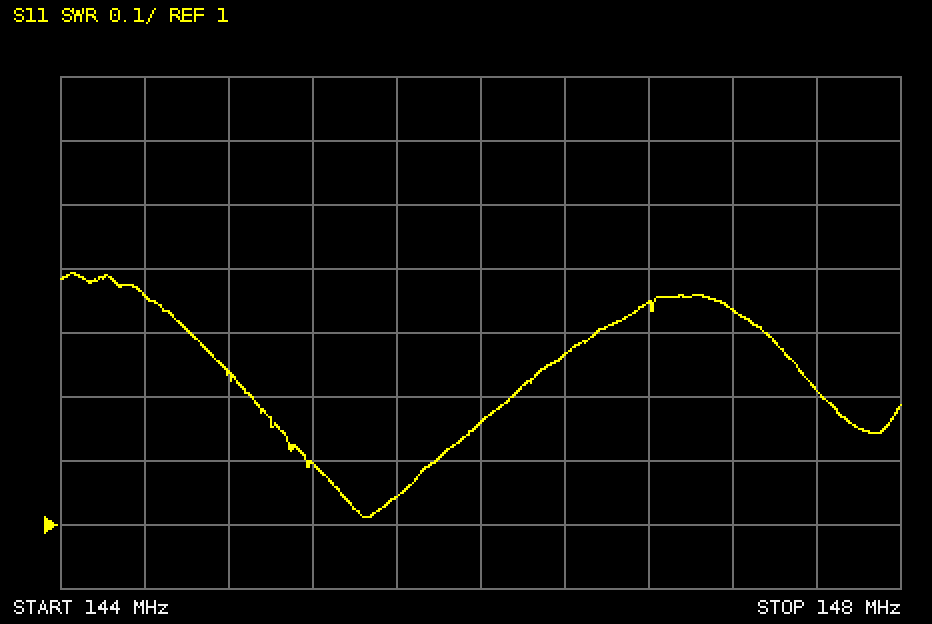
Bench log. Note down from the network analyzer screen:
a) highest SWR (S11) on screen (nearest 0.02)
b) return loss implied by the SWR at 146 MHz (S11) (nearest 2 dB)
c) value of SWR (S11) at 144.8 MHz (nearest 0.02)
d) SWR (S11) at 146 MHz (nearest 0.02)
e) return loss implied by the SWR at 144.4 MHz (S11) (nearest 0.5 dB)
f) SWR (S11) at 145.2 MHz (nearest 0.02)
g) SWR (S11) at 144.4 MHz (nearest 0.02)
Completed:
1.40
22 dB
1.24
1.16
16.5 dB
1.10
1.36
